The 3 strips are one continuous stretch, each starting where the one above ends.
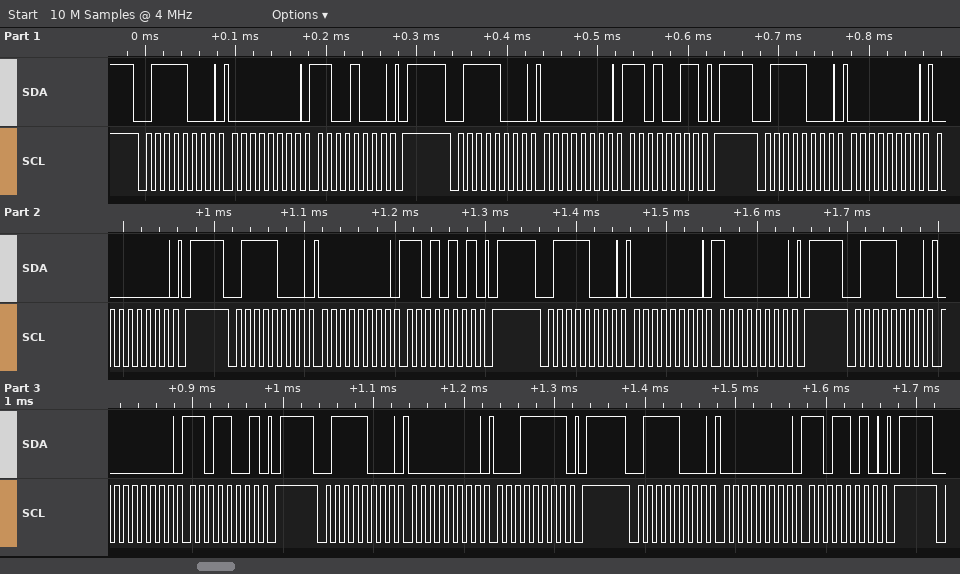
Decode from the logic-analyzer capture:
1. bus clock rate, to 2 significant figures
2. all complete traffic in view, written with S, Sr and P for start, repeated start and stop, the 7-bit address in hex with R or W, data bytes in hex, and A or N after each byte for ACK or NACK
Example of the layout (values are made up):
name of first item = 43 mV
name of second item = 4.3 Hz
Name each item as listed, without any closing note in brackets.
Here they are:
bus clock rate, to 2 significant figures = 100 kHz
all complete traffic in view, written with S, Sr and P for start, repeated start and stop, the 7-bit address in hex with R or W, data bytes in hex, and A or N after each byte for ACK or NACK = S 3CW A 00 A C8 A P S 3CW A 00 A D3 A P S 3CW A 00 A 00 A P S 3CW A 00 A D5 A P S 3CW A 00 A 80 A P S 3CW A 00 A D9 A P S 3CW A 00 A 1F A P S 3CW A 00 A DA A P
